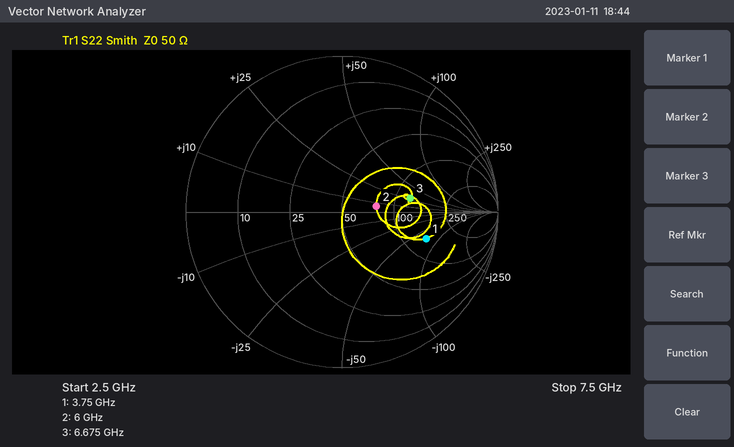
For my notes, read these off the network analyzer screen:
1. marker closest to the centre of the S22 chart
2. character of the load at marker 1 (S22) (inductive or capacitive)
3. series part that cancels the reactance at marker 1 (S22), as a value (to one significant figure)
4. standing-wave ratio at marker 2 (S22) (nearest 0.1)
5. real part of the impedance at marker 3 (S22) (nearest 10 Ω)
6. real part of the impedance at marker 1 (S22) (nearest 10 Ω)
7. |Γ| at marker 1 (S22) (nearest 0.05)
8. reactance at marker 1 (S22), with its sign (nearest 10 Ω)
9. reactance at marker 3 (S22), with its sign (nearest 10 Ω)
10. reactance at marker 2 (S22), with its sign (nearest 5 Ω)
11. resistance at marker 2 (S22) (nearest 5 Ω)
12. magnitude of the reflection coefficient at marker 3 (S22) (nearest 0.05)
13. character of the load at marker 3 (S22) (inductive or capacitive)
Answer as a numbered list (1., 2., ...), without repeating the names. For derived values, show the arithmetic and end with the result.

1. marker 2
2. capacitive
3. L = 70 Ω/(2π × 3.75 GHz) ≈ 3 nH
4. 1.6
5. 120 Ω
6. 140 Ω
7. 0.55
8. -70 Ω
9. +30 Ω
10. +5 Ω
11. 80 Ω
12. 0.45
13. inductive
